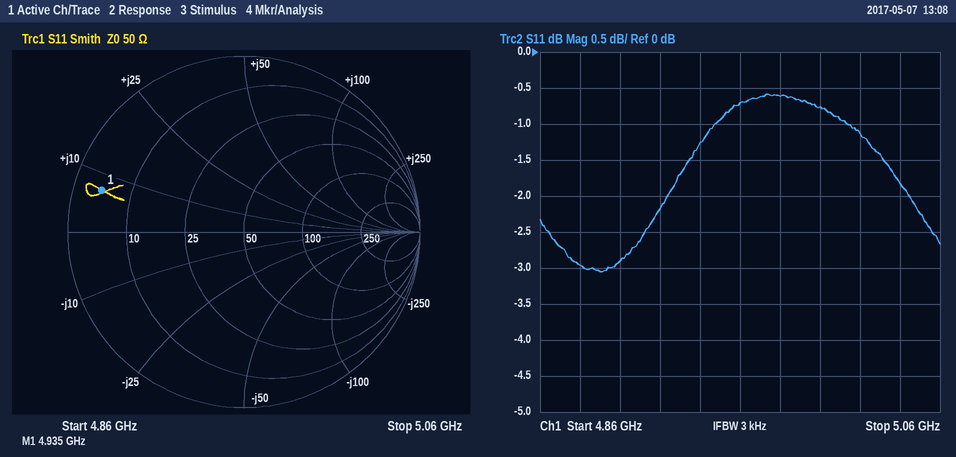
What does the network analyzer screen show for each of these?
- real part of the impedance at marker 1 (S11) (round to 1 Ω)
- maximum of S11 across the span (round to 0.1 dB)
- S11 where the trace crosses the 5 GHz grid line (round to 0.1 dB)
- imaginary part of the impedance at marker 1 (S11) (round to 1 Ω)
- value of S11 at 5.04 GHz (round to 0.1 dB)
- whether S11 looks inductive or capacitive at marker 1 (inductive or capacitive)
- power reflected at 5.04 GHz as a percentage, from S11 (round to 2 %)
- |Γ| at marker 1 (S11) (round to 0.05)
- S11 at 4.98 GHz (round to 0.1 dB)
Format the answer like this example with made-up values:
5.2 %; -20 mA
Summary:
4 Ω; -0.6 dB; -0.8 dB; +7 Ω; -1.8 dB; inductive; 66 %; 0.85; -0.6 dB
